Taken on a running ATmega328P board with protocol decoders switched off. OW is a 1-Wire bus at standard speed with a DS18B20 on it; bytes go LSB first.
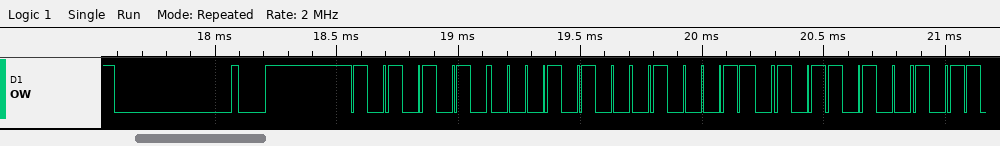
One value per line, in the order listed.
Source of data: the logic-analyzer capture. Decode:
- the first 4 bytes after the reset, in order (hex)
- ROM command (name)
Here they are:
55 28 62 2D
Match ROM
